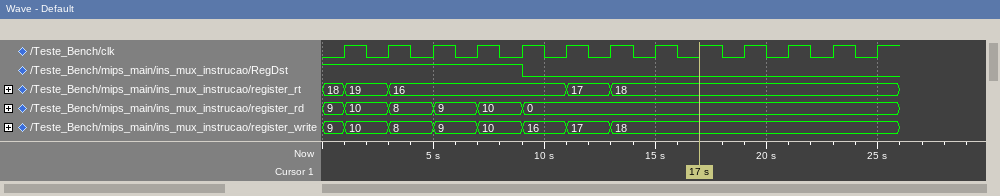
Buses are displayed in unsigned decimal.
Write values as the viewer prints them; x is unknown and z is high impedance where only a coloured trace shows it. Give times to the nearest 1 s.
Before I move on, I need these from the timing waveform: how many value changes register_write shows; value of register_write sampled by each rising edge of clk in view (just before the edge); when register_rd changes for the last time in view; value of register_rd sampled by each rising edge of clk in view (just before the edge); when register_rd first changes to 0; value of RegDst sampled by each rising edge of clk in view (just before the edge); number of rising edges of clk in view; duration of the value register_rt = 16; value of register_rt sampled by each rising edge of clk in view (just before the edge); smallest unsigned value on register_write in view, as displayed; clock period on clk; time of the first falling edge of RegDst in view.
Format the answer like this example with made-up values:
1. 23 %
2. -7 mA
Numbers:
1. 7
2. 9, 10, 8, 9, 10, 16, 17, 18, 18, 18, 18, 18, 18
3. 9 s
4. 9, 10, 8, 9, 10, 0, 0, 0, 0, 0, 0, 0, 0
5. 9 s
6. 1 1 1 1 1 0 0 0 0 0 0 0 0
7. 13
8. 8 s
9. 18, 19, 16, 16, 16, 16, 17, 18, 18, 18, 18, 18, 18
10. 8
11. 2 s
12. 9 s
